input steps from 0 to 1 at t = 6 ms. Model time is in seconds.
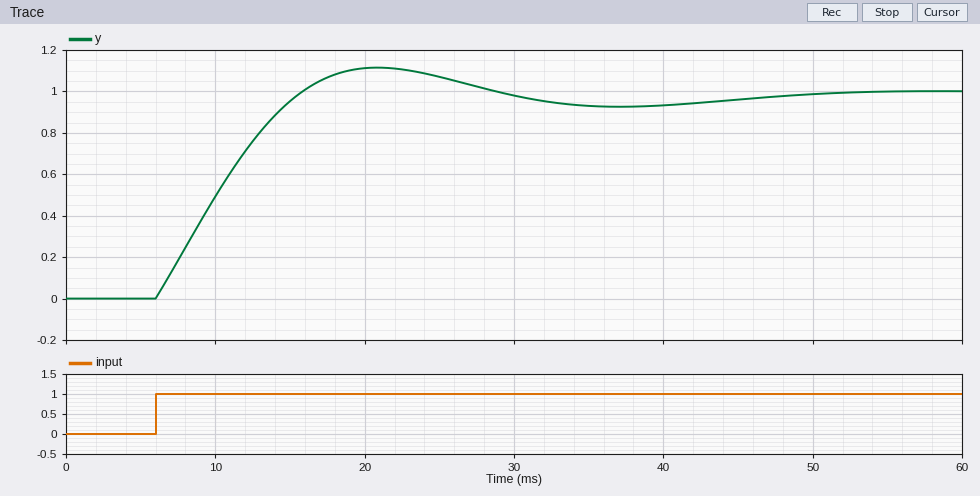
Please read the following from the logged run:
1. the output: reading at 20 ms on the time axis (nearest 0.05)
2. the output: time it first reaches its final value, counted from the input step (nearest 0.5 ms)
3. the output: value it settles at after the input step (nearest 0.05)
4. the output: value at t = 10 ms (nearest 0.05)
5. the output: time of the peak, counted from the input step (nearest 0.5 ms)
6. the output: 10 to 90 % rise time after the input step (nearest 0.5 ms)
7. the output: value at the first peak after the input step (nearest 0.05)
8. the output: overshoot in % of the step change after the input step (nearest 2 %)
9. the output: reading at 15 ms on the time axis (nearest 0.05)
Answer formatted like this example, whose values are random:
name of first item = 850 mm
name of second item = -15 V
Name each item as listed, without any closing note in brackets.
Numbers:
the output: reading at 20 ms on the time axis = 1.10
the output: time it first reaches its final value, counted from the input step = 10.0 ms
the output: value it settles at after the input step = 1.00
the output: value at t = 10 ms = 0.50
the output: time of the peak, counted from the input step = 15.0 ms
the output: 10 to 90 % rise time after the input step = 7.5 ms
the output: value at the first peak after the input step = 1.10
the output: overshoot in % of the step change after the input step = 12 %
the output: reading at 15 ms on the time axis = 0.95
